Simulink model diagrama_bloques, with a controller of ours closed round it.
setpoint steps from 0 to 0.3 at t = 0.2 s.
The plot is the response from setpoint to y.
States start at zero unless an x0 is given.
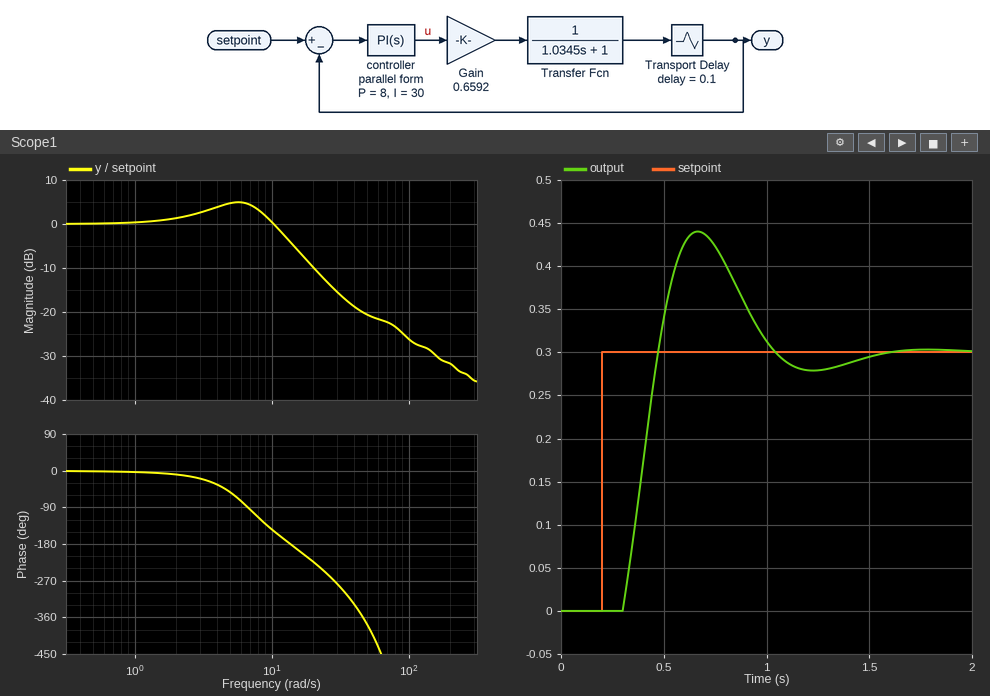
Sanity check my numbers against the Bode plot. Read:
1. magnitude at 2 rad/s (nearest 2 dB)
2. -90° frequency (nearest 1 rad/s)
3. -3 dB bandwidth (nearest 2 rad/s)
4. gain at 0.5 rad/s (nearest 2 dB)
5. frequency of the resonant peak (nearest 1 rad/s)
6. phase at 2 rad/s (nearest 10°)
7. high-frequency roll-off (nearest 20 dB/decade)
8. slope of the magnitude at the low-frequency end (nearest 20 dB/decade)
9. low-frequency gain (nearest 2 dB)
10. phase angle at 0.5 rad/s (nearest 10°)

2 dB
7 rad/s
12 rad/s
0 dB
6 rad/s
-10°
-20 dB/decade
0 dB/decade
0 dB
0°
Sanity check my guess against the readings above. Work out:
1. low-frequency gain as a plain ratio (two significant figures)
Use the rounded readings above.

1.0
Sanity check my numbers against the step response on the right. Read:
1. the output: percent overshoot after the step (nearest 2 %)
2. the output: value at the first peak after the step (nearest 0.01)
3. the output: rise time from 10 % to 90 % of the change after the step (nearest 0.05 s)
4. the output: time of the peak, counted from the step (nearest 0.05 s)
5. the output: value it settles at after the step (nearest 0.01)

46 %
0.44
0.15 s
0.45 s
0.30
